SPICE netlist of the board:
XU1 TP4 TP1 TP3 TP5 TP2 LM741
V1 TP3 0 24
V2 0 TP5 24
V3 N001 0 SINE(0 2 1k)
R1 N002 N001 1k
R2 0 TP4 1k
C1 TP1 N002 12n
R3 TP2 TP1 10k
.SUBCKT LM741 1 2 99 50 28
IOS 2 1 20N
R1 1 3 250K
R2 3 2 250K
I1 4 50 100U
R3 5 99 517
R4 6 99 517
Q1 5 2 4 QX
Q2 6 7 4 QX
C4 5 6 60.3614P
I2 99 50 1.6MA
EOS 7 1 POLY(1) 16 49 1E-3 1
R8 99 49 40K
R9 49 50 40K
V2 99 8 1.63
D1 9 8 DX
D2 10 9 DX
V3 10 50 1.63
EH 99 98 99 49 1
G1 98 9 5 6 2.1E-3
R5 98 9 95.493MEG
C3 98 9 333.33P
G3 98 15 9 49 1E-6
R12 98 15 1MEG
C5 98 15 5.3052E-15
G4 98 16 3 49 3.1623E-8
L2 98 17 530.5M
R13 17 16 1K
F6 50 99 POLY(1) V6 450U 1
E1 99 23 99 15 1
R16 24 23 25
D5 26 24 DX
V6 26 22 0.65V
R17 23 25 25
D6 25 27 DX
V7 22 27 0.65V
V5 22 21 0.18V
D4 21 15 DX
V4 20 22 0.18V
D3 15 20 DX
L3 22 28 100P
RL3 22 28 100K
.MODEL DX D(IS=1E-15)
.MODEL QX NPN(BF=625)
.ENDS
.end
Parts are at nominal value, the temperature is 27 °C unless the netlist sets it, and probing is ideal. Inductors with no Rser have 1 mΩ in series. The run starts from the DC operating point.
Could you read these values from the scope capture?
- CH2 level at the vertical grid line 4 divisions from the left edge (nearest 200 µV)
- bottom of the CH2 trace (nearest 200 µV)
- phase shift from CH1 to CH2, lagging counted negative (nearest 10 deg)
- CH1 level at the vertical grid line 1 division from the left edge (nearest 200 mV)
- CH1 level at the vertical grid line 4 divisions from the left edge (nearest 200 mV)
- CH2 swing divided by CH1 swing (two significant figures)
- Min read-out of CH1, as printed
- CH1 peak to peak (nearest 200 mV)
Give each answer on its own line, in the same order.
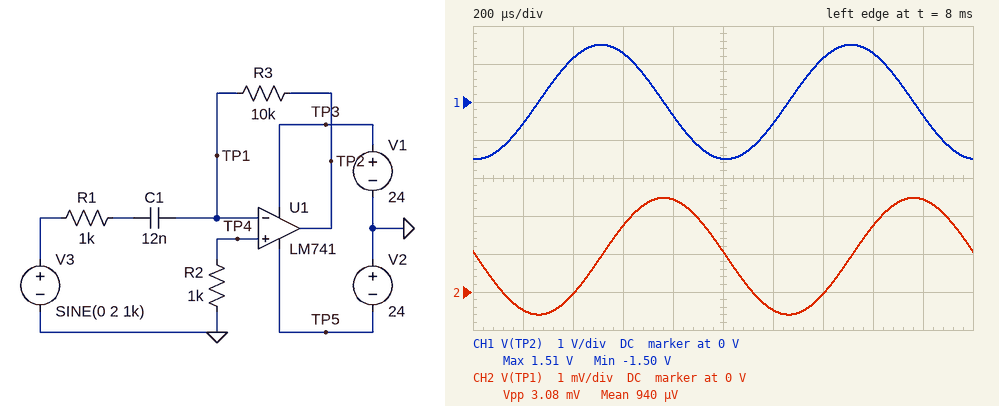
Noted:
2.4 mV
-600 µV
-90 deg
-600 mV
-400 mV
0.0010
-1.50 V
3.0 V
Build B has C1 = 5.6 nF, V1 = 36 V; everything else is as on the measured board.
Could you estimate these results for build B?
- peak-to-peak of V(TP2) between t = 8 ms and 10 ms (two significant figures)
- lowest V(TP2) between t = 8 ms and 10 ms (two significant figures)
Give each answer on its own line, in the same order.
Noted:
1.4 V
-700 mV
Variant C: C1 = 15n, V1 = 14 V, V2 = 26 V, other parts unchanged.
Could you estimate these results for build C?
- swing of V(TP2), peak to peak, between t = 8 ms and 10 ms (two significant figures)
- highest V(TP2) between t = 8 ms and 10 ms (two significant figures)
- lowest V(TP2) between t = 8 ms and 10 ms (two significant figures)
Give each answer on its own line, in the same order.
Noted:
3.8 V
1.9 V
-1.9 V
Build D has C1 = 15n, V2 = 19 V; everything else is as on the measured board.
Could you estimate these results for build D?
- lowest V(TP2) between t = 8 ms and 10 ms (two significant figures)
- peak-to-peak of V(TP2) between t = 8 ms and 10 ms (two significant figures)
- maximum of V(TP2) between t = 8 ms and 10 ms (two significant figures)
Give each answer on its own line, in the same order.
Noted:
-1.9 V
3.8 V
1.9 V
